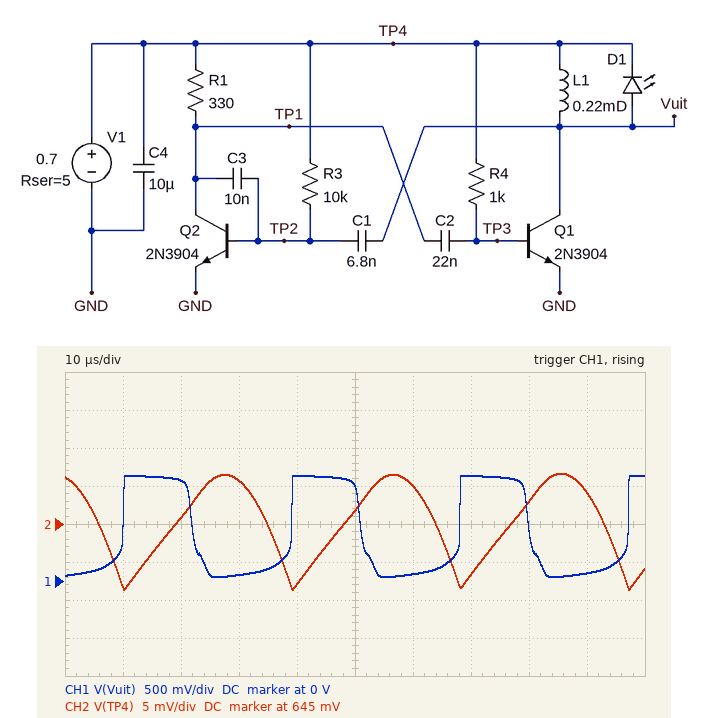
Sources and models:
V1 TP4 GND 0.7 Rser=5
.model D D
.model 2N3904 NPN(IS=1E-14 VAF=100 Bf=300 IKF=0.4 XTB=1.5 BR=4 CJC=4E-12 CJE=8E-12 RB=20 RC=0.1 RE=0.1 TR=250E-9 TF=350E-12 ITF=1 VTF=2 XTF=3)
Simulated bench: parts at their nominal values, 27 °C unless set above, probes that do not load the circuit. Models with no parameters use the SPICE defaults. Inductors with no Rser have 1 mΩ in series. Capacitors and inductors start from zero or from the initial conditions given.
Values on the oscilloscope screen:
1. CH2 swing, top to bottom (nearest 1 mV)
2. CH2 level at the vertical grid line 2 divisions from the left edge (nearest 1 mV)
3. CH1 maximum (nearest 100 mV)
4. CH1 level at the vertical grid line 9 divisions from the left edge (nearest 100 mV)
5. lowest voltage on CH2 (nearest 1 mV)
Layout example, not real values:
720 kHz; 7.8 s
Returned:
15 mV; 646 mV; 1.4 V; 100 mV; 636 mV
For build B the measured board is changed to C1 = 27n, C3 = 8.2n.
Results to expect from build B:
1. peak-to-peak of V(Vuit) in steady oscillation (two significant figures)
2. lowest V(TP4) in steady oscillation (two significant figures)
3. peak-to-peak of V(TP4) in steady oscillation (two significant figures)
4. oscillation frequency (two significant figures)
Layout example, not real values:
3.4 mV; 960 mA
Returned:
1.3 V; 610 mV; 25 mV; 26 kHz
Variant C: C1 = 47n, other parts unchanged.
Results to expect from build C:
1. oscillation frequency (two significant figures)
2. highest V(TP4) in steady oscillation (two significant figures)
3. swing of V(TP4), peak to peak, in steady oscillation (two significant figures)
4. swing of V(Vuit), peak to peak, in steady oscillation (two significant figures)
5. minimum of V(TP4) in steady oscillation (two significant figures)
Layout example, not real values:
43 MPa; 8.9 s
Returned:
23 kHz; 630 mV; 29 mV; 1.2 V; 600 mV
